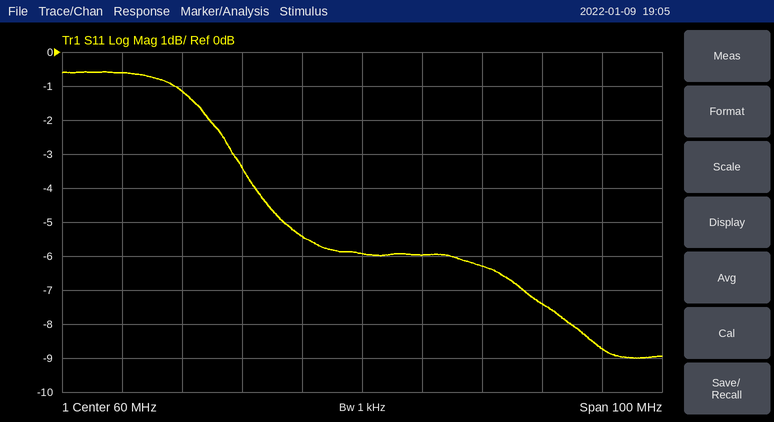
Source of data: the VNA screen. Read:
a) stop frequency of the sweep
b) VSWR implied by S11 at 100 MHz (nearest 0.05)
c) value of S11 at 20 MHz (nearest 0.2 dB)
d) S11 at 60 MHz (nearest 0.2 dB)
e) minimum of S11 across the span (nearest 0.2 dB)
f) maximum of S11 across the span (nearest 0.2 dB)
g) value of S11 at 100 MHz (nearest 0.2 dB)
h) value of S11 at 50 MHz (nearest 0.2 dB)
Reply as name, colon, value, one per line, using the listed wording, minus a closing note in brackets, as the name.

stop frequency of the sweep: 110 MHz
VSWR implied by S11 at 100 MHz: 2.15
value of S11 at 20 MHz: -0.6 dB
S11 at 60 MHz: -6.0 dB
minimum of S11 across the span: -9.0 dB
maximum of S11 across the span: -0.6 dB
value of S11 at 100 MHz: -8.8 dB
value of S11 at 50 MHz: -5.4 dB
